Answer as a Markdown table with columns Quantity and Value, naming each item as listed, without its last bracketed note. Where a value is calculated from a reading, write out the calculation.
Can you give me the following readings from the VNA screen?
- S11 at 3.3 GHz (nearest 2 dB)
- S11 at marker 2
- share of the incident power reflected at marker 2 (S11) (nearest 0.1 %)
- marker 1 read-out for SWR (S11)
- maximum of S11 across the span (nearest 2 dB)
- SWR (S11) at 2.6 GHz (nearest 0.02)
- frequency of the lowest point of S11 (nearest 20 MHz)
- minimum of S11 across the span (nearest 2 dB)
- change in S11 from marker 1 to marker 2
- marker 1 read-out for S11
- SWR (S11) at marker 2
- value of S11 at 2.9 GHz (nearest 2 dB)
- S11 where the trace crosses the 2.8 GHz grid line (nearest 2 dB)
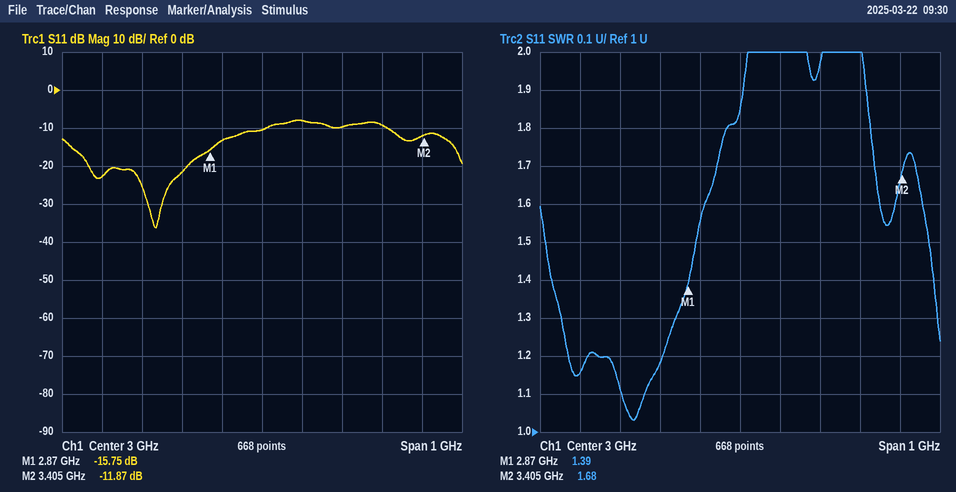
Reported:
| Quantity | Value |
|---|---|
| S11 at 3.3 GHz | -10 dB |
| S11 at marker 2 | -11.87 dB |
| share of the incident power reflected at marker 2 (S11) | 10^(-11.87/10) ≈ 6.5 % |
| marker 1 read-out for SWR | 1.39 |
| maximum of S11 across the span | -8 dB |
| SWR (S11) at 2.6 GHz | 1.16 |
| frequency of the lowest point of S11 | 2.74 GHz |
| minimum of S11 across the span | -36 dB |
| change in S11 from marker 1 to marker 2 | -11.87 − (-15.75) = 3.88 dB |
| marker 1 read-out for S11 | -15.75 dB |
| SWR (S11) at marker 2 | 1.68 |
| value of S11 at 2.9 GHz | -14 dB |
| S11 where the trace crosses the 2.8 GHz grid line | -22 dB |
